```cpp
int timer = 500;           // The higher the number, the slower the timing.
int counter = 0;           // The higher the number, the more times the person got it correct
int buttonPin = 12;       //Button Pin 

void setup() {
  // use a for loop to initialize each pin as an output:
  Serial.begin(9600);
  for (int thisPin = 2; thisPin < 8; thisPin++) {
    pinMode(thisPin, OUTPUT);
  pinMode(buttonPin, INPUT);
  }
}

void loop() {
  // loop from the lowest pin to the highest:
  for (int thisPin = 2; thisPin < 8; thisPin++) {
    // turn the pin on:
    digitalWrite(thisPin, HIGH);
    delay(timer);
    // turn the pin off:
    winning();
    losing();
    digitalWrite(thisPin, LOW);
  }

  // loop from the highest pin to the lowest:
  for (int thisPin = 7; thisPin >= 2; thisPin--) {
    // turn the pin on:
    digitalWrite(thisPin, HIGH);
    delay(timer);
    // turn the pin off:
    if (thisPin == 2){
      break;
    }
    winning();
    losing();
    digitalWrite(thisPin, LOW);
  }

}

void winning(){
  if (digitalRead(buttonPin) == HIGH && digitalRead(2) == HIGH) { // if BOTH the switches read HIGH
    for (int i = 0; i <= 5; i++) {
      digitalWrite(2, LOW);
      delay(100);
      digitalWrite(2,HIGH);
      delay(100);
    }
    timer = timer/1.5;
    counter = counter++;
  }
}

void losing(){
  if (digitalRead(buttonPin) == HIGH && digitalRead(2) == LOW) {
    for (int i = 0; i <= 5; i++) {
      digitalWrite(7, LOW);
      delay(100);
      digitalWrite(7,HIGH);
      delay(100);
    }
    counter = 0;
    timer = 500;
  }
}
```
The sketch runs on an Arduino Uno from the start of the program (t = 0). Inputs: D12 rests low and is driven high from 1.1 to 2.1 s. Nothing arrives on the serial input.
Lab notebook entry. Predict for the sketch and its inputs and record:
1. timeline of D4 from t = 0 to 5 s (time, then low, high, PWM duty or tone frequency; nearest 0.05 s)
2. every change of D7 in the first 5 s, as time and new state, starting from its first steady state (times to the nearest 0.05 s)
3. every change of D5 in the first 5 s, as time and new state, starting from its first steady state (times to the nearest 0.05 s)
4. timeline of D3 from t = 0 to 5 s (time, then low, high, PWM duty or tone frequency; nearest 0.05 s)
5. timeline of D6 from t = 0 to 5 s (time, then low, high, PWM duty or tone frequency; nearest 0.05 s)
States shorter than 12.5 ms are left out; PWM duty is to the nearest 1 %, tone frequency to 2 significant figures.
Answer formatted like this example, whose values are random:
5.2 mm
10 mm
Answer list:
0 s low; 1 s high; 2.7 s low
0 s low; 1.6 s high; 1.7 s low; 1.8 s high; 1.9 s low; 2 s high; 2.1 s low; 2.2 s high; 2.3 s low; 2.4 s high; 2.5 s low; 2.6 s high; 4.7 s low
0 s low; 2.7 s high; 3.2 s low
0 s low; 0.5 s high; 1 s low
0 s low; 3.2 s high; 3.7 s low; 4.7 s high
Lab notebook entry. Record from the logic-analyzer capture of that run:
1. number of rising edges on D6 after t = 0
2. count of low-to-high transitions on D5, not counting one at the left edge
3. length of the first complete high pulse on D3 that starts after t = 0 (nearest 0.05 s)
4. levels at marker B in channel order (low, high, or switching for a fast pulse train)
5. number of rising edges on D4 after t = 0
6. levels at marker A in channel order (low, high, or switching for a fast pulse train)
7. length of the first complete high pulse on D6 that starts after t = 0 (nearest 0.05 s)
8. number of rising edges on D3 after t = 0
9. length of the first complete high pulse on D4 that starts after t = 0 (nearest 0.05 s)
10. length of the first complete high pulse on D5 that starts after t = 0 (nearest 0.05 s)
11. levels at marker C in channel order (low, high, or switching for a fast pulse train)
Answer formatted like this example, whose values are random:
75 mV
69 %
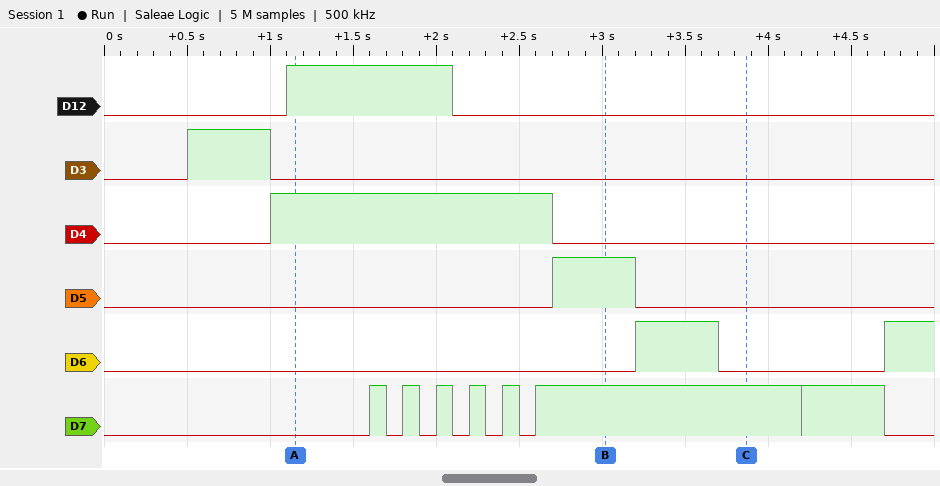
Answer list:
2
1
0.50 s
D12 low, D3 low, D4 low, D5 high, D6 low, D7 high
1
D12 high, D3 low, D4 high, D5 low, D6 low, D7 low
0.50 s
1
1.70 s
0.50 s
D12 low, D3 low, D4 low, D5 low, D6 low, D7 high
